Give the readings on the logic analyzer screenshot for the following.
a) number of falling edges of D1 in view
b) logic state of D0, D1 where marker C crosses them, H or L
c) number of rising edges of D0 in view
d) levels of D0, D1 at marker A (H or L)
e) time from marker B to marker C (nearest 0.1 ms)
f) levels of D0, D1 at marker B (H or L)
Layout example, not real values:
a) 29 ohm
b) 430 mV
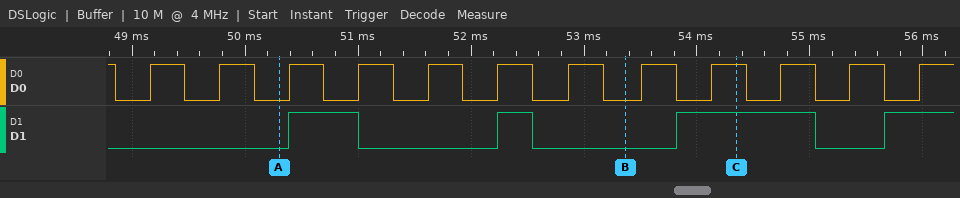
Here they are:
a) 3
b) D0=H, D1=H
c) 12
d) D0=L, D1=L
e) 1 ms
f) D0=L, D1=L
